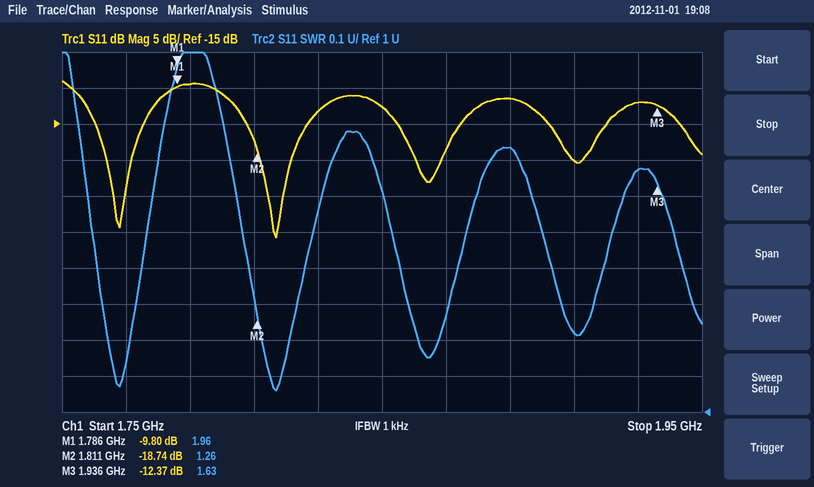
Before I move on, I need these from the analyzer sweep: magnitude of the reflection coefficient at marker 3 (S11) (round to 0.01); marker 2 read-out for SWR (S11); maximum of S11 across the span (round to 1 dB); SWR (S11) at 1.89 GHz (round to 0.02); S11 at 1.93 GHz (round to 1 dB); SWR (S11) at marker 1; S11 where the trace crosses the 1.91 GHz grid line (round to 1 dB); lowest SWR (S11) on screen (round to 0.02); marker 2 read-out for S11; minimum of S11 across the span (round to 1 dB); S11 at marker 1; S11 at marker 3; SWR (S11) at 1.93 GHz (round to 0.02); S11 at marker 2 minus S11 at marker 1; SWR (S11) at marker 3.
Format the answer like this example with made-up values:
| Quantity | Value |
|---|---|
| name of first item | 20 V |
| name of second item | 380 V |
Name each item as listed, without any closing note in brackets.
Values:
| Quantity | Value |
|---|---|
| magnitude of the reflection coefficient at marker 3 (S11) | 0.24 |
| marker 2 read-out for SWR | 1.26 |
| maximum of S11 across the span | -9 dB |
| SWR (S11) at 1.89 GHz | 1.74 |
| S11 at 1.93 GHz | -12 dB |
| SWR (S11) at marker 1 | 1.96 |
| S11 where the trace crosses the 1.91 GHz grid line | -20 dB |
| lowest SWR (S11) on screen | 1.06 |
| marker 2 read-out for S11 | -18.74 dB |
| minimum of S11 across the span | -31 dB |
| S11 at marker 1 | -9.80 dB |
| S11 at marker 3 | -12.37 dB |
| SWR (S11) at 1.93 GHz | 1.68 |
| S11 at marker 2 minus S11 at marker 1 | -8.94 dB |
| SWR (S11) at marker 3 | 1.63 |
